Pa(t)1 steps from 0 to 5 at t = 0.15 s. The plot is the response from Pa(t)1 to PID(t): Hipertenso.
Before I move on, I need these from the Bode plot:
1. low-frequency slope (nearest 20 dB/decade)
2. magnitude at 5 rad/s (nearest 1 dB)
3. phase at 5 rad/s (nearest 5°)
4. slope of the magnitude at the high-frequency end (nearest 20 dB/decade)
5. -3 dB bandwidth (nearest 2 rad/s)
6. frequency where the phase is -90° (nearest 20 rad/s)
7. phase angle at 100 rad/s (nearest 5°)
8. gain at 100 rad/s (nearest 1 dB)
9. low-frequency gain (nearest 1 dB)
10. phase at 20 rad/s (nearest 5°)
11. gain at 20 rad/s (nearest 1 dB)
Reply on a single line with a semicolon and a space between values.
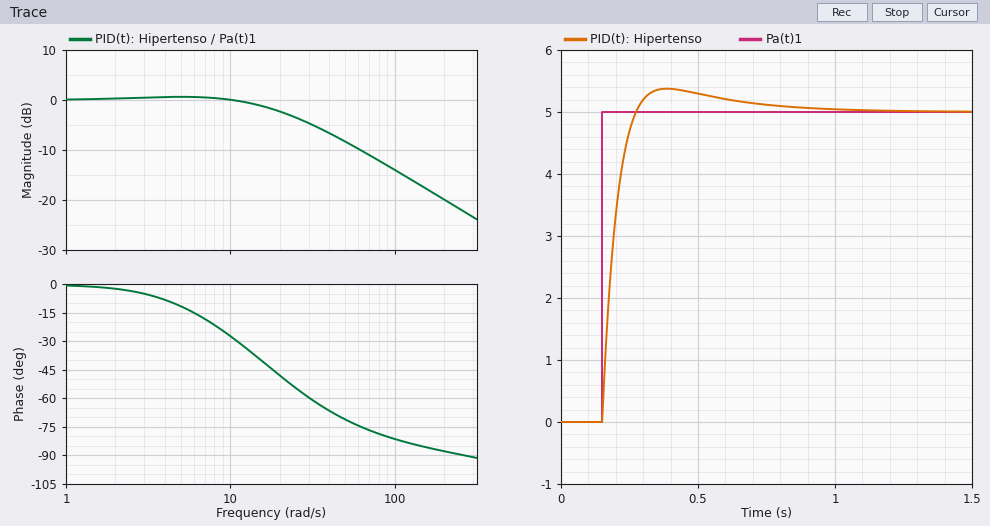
0 dB/decade; 1 dB; -10°; -20 dB/decade; 22 rad/s; 260 rad/s; -80°; -14 dB; 0 dB; -50°; -2 dB
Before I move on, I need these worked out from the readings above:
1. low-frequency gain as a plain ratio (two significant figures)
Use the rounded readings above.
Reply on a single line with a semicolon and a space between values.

1.0
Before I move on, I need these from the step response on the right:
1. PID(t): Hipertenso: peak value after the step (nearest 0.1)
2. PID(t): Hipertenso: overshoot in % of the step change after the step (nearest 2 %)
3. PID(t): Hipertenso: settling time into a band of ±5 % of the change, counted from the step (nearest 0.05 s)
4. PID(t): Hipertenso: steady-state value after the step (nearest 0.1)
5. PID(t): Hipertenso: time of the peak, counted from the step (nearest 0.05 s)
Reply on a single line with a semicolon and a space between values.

5.4; 8 %; 0.40 s; 5.0; 0.25 s
